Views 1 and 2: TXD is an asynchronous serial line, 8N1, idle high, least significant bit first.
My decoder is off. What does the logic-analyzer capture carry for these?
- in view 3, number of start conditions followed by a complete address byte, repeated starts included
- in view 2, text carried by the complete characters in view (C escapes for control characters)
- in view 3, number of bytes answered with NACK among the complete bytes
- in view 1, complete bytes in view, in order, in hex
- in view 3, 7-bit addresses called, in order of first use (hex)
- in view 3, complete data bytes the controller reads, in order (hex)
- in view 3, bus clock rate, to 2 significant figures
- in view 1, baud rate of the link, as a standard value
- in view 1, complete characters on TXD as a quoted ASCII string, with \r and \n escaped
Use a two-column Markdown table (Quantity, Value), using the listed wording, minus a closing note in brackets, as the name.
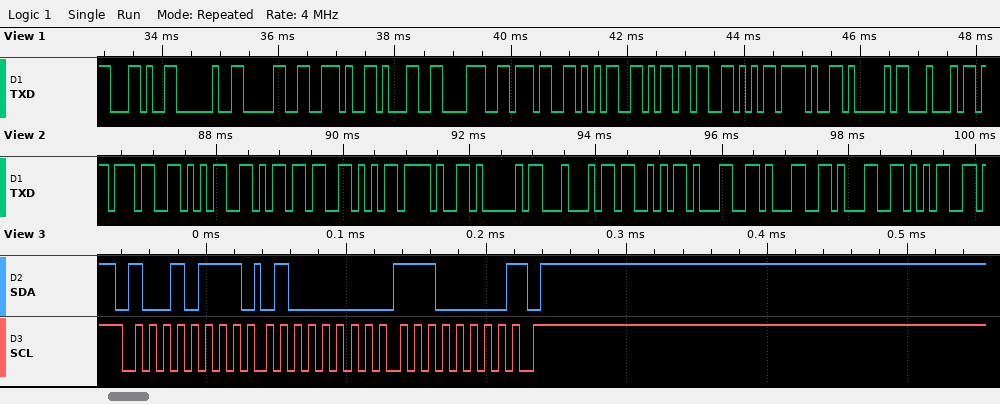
| Quantity | Value |
|---|---|
| in view 3, number of start conditions followed by a complete address byte, repeated starts included | 1 |
| in view 2, text carried by the complete characters in view | "75mV/ADS1115" |
| in view 3, number of bytes answered with NACK among the complete bytes | 1 |
| in view 1, complete bytes in view, in order, in hex | 2C 20 30 2E 31 38 37 35 6D 56 2F 41 44 |
| in view 3, 7-bit addresses called, in order of first use | 0x4B |
| in view 3, complete data bytes the controller reads, in order | 40 E0 |
| in view 3, bus clock rate, to 2 significant figures | 100 kHz |
| in view 1, baud rate of the link, as a standard value | 9600 baud |
| in view 1, complete characters on TXD as a quoted ASCII string, with \r and \n escaped | ", 0.1875mV/AD" |
